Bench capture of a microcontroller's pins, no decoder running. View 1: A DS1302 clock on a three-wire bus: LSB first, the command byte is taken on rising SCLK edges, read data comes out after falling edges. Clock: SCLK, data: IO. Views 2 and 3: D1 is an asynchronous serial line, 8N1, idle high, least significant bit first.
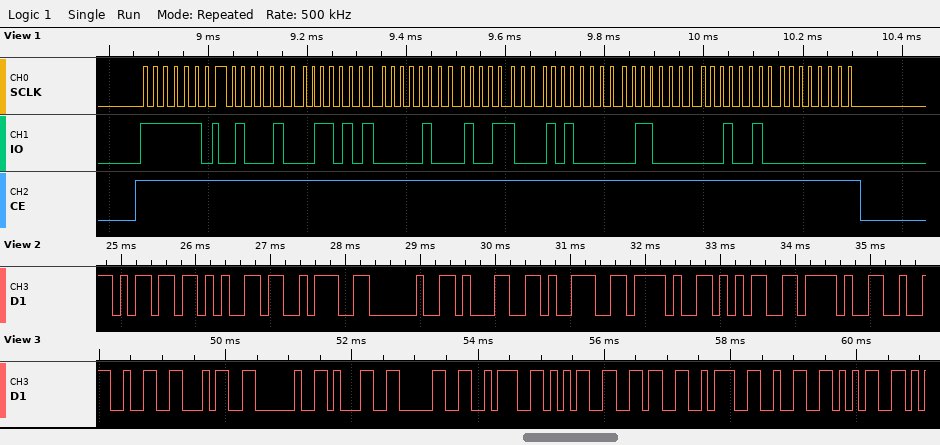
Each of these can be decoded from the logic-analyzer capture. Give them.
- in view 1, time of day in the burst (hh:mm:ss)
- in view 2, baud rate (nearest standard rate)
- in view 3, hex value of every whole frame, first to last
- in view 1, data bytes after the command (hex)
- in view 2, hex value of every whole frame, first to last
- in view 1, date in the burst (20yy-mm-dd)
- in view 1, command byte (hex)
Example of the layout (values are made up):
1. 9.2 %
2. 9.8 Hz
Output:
1. 10:56:22
2. 9600 baud
3. 32 34 20 31 30 3A 35 36 3A 32 35
4. 22 56 10 19 05 06 24 00
5. 0x6D 0x65 0x3A 0x20 0x31 0x39 0x2F 0x35 0x2F
6. 2024-05-19
7. 0xBF
